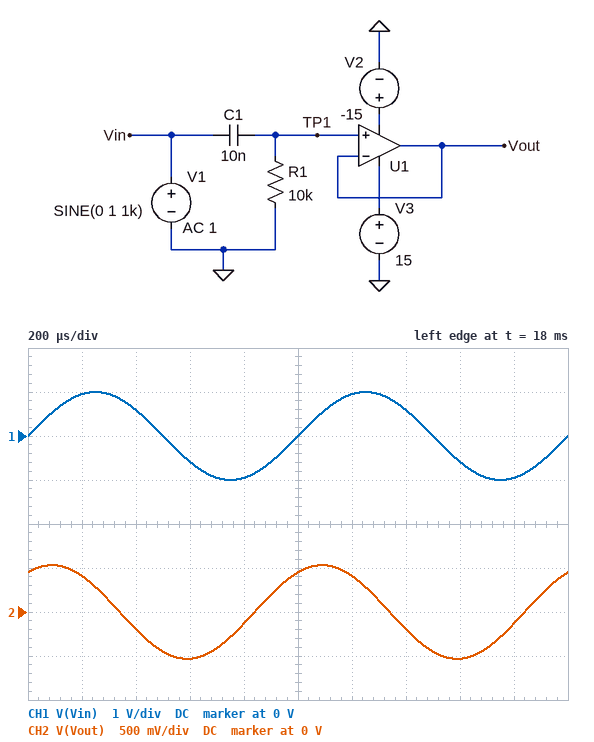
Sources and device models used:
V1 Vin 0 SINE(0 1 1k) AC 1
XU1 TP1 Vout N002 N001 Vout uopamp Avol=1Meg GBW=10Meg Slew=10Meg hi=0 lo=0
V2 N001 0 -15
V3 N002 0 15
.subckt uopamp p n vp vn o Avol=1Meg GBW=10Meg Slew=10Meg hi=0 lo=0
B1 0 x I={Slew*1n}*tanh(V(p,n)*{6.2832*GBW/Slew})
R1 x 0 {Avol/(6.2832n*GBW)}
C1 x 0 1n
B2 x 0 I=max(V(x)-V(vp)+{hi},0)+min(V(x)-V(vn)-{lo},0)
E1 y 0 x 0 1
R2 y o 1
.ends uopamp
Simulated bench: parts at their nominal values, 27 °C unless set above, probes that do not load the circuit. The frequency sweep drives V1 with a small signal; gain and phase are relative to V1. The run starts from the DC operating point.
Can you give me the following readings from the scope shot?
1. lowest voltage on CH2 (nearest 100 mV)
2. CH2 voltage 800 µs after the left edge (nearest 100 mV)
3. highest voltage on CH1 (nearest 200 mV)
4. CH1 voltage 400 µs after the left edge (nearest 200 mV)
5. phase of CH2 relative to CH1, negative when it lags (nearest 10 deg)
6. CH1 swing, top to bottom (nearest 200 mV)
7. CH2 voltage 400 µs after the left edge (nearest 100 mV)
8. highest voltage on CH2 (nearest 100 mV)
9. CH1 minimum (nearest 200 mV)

-500 mV
-100 mV
1.0 V
600 mV
60 deg
2.0 V
-200 mV
500 mV
-1.0 V
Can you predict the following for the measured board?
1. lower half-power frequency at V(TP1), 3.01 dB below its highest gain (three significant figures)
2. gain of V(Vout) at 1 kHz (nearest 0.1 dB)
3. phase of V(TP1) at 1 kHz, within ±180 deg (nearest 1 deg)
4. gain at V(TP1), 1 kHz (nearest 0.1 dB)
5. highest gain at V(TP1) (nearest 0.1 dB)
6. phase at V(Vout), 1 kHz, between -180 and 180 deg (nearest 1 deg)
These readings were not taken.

1.59 kHz
-5.5 dB
58 deg
-5.5 dB
0 dB
58 deg
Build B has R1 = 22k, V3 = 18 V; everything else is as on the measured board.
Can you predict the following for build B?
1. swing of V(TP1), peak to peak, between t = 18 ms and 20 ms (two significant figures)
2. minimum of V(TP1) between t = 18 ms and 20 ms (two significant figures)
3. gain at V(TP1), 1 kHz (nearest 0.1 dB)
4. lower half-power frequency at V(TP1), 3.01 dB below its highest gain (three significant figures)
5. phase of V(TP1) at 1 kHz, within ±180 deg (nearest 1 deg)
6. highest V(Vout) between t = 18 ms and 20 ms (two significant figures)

1.6 V
-810 mV
-1.8 dB
723 Hz
36 deg
810 mV
